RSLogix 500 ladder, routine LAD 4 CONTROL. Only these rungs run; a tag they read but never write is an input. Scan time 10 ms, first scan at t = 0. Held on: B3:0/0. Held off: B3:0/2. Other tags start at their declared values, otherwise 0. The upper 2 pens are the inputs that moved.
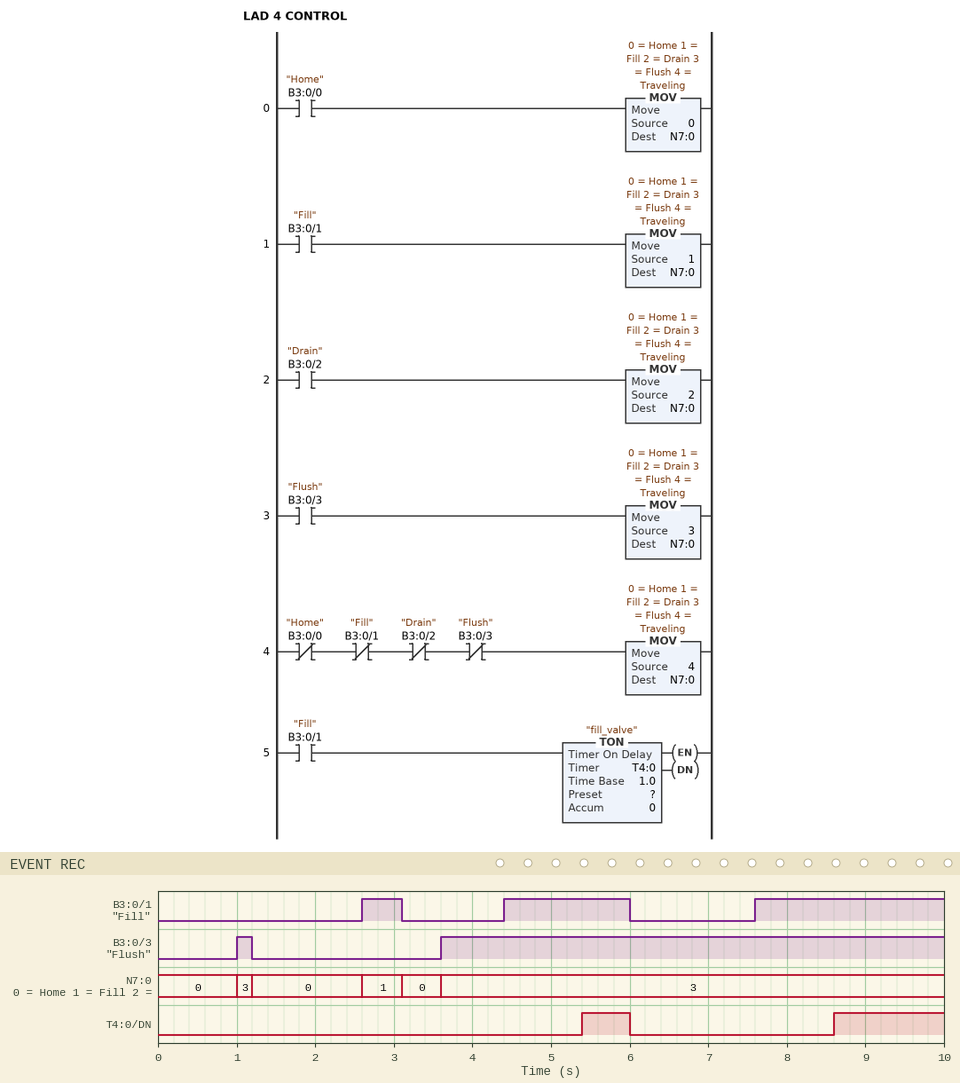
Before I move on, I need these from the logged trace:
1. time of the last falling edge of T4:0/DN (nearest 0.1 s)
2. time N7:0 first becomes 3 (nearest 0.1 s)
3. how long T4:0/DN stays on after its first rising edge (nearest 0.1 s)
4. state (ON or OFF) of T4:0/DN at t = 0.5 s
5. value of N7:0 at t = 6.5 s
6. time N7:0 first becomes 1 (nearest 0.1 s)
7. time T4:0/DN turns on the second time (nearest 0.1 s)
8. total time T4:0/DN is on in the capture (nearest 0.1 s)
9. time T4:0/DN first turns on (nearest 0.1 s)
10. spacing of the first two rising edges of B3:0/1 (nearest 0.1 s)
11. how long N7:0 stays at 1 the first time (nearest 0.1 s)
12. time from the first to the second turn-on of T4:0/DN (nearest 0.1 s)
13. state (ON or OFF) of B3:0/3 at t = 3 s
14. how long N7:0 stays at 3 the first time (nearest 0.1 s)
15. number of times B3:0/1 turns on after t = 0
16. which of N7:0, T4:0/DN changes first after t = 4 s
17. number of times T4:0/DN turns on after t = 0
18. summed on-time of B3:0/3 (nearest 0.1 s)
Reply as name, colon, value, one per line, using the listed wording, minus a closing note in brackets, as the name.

time of the last falling edge of T4:0/DN: 6.0 s
time N7:0 first becomes 3: 1.0 s
how long T4:0/DN stays on after its first rising edge: 0.6 s
state (ON or OFF) of T4:0/DN at t = 0.5 s: OFF
value of N7:0 at t = 6.5 s: 3
time N7:0 first becomes 1: 2.6 s
time T4:0/DN turns on the second time: 8.6 s
total time T4:0/DN is on in the capture: 2.0 s
time T4:0/DN first turns on: 5.4 s
spacing of the first two rising edges of B3:0/1: 1.8 s
how long N7:0 stays at 1 the first time: 0.5 s
time from the first to the second turn-on of T4:0/DN: 3.2 s
state (ON or OFF) of B3:0/3 at t = 3 s: OFF
how long N7:0 stays at 3 the first time: 0.2 s
number of times B3:0/1 turns on after t = 0: 3
which of N7:0, T4:0/DN changes first after t = 4 s: T4:0/DN
number of times T4:0/DN turns on after t = 0: 2
summed on-time of B3:0/3: 6.6 s
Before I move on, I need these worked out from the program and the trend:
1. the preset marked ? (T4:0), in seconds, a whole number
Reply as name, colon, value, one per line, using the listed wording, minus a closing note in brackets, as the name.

the preset marked ? (T4:0), in seconds, a whole number: 1 s
